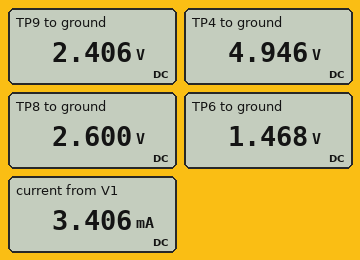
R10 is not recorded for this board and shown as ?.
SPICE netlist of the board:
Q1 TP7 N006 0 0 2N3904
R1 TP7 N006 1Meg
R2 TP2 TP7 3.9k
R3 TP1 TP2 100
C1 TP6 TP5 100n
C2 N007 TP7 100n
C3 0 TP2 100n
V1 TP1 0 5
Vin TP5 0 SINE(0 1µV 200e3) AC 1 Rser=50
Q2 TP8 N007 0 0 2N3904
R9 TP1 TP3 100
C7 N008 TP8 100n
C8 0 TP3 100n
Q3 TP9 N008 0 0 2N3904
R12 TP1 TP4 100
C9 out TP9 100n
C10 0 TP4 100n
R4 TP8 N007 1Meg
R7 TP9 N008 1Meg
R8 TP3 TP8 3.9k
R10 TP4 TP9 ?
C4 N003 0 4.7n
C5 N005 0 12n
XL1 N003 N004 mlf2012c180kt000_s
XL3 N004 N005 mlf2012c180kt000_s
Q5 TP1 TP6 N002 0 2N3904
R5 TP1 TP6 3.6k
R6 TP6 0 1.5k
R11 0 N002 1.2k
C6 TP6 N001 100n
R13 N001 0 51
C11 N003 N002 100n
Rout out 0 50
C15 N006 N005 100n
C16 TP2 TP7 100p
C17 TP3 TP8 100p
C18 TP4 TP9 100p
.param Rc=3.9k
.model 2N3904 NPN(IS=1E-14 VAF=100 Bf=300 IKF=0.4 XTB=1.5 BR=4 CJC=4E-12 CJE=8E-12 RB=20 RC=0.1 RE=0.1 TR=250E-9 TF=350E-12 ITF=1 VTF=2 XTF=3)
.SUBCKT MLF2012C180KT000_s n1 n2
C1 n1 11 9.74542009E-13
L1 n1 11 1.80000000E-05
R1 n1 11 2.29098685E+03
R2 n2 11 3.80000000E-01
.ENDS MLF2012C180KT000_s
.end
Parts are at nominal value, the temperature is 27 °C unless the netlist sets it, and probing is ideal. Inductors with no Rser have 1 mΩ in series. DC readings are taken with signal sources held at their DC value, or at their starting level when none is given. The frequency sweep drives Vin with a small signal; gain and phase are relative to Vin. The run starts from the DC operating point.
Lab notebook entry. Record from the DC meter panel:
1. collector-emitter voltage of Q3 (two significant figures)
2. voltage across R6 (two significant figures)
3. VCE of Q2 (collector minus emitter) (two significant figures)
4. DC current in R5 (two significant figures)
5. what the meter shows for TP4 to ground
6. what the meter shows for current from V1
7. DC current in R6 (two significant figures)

2.4 V
1.5 V
2.6 V
980 µA
4.946 V
3.406 mA
980 µA
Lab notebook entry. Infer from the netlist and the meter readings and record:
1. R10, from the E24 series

4.7 kΩ
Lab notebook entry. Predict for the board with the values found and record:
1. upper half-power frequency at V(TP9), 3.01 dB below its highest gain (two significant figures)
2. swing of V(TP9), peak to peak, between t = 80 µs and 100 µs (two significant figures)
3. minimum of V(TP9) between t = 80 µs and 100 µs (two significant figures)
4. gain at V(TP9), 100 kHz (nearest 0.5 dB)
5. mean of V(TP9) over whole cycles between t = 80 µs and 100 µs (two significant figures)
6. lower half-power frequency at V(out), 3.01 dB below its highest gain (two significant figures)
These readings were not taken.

1.6 kHz
3.1 mV
2.4 V
64.0 dB
2.4 V
980 Hz
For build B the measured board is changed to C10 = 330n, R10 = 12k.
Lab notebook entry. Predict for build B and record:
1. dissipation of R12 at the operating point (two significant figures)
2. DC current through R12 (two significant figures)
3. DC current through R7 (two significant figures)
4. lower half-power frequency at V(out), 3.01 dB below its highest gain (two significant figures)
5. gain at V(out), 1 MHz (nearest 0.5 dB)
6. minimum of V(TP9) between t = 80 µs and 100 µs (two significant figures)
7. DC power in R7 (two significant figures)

8.1 µW
280 µA
940 nA
870 Hz
15.5 dB
1.6 V
880 nW
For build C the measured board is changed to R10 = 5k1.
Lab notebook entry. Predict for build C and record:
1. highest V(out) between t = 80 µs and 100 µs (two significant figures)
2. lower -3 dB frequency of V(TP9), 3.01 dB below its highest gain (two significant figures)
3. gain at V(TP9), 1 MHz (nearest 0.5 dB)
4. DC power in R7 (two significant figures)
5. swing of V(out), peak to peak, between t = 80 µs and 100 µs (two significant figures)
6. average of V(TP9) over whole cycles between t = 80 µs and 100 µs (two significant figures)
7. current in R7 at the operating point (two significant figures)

1.4 mV
360 Hz
20.5 dB
2.8 µW
2.9 mV
2.3 V
1.7 µA
